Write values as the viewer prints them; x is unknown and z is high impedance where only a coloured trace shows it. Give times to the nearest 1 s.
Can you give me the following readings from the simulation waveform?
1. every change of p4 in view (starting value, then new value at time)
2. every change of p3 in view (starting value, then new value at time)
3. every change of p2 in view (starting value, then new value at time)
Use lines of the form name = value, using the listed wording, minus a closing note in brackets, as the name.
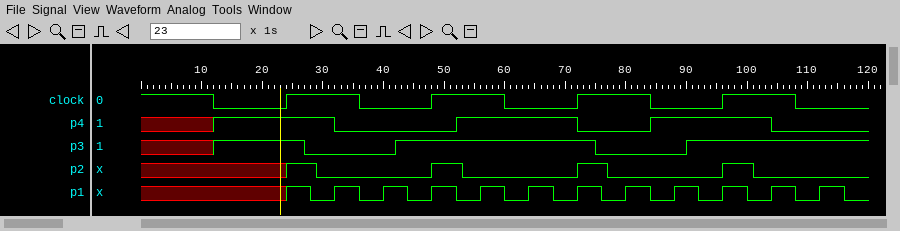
every change of p4 in view = x, 1 at 12 s, 0 at 32 s, 1 at 52 s, 0 at 72 s, 1 at 84 s, 0 at 104 s
every change of p3 in view = x, 1 at 12 s, 0 at 27 s, 1 at 42 s, 0 at 75 s, 1 at 90 s
every change of p2 in view = x, 1 at 24 s, 0 at 29 s, 1 at 48 s, 0 at 53 s, 1 at 72 s, 0 at 77 s, 1 at 96 s, 0 at 101 s
